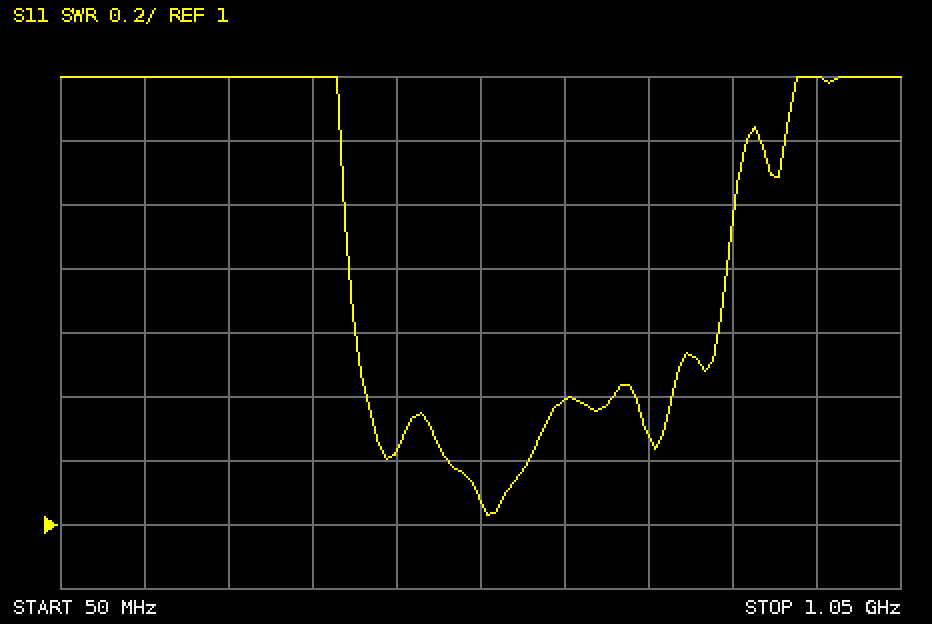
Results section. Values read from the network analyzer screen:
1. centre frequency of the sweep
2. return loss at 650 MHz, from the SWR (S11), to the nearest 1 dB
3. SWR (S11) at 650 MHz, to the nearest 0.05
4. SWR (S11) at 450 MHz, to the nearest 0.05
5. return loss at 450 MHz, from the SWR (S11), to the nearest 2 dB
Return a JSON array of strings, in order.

["550 MHz", "16 dB", "1.40", "1.25", "20 dB"]
